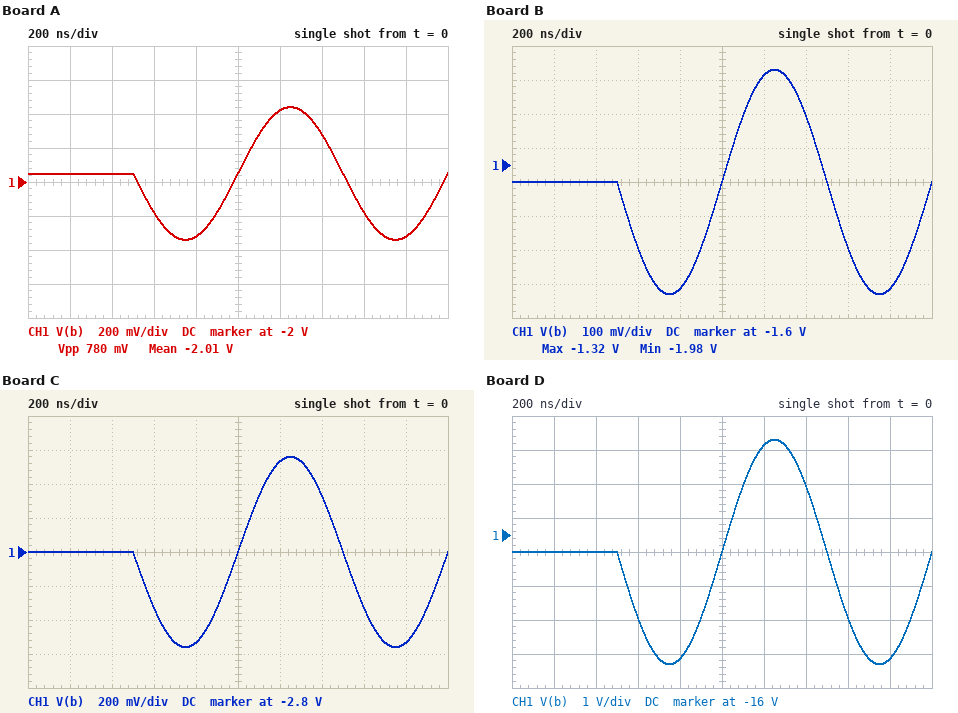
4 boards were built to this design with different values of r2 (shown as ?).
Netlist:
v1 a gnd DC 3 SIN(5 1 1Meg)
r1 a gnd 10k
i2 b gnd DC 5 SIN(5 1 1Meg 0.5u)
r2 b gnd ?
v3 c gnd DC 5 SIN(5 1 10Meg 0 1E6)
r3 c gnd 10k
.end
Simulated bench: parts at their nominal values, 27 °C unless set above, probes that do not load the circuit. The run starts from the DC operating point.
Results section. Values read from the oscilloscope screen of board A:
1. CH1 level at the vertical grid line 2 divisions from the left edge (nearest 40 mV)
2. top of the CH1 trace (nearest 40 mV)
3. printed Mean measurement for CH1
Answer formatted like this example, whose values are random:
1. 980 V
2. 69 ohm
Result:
1. -1.96 V
2. -1.56 V
3. -2.01 V
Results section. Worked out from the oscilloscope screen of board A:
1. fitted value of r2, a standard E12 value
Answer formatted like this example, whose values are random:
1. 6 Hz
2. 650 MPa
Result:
1. 0.39 Ω
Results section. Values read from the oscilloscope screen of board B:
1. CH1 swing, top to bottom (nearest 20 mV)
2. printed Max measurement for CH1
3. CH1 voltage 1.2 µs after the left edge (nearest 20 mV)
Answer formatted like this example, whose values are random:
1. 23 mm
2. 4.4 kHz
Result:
1. 660 mV
2. -1.32 V
3. -1.34 V
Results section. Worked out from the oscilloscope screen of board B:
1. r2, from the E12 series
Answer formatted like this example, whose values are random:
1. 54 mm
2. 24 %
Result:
1. 0.33 Ω
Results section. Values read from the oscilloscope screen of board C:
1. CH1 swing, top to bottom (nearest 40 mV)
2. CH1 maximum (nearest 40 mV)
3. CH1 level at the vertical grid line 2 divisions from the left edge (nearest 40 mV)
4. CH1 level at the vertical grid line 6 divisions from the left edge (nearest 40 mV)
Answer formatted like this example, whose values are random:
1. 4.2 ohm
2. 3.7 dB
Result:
1. 1.12 V
2. -2.24 V
3. -2.80 V
4. -2.28 V
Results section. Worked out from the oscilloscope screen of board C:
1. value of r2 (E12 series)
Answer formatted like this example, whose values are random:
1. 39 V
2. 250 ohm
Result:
1. 0.56 Ω
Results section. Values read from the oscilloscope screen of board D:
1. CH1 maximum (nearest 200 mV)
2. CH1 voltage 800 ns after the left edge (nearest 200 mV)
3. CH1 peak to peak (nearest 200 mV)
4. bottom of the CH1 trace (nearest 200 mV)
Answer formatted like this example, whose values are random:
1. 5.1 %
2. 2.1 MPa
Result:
1. -13.2 V
2. -19.6 V
3. 6.6 V
4. -19.8 V
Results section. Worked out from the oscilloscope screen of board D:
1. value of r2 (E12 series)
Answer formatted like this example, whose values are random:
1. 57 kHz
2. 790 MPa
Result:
1. 3.3 Ω
